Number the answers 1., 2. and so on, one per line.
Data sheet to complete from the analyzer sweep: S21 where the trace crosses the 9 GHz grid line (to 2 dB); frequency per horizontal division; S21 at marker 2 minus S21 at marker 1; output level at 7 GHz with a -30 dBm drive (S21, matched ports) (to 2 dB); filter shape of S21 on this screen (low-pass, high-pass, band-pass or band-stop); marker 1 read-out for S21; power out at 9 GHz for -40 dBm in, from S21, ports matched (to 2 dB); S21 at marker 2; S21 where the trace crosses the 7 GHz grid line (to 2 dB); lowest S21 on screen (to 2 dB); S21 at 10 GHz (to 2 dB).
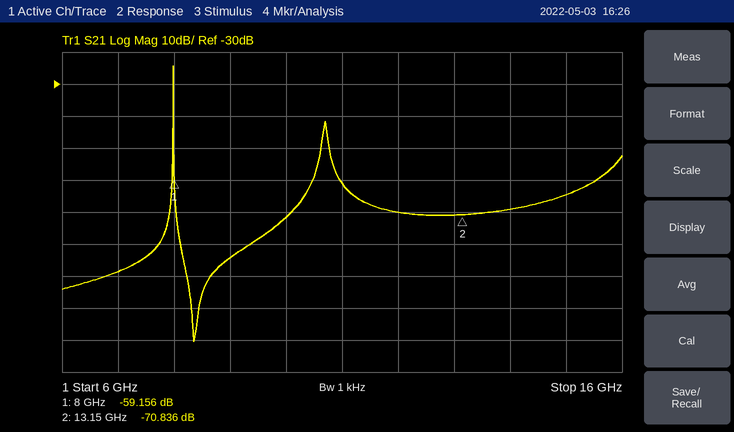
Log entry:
1. -84 dB
2. 1 GHz
3. -11.680 dB
4. -118 dBm
5. band-pass
6. -59.156 dB
7. -124 dBm
8. -70.836 dB
9. -88 dB
10. -110 dB
11. -72 dB
